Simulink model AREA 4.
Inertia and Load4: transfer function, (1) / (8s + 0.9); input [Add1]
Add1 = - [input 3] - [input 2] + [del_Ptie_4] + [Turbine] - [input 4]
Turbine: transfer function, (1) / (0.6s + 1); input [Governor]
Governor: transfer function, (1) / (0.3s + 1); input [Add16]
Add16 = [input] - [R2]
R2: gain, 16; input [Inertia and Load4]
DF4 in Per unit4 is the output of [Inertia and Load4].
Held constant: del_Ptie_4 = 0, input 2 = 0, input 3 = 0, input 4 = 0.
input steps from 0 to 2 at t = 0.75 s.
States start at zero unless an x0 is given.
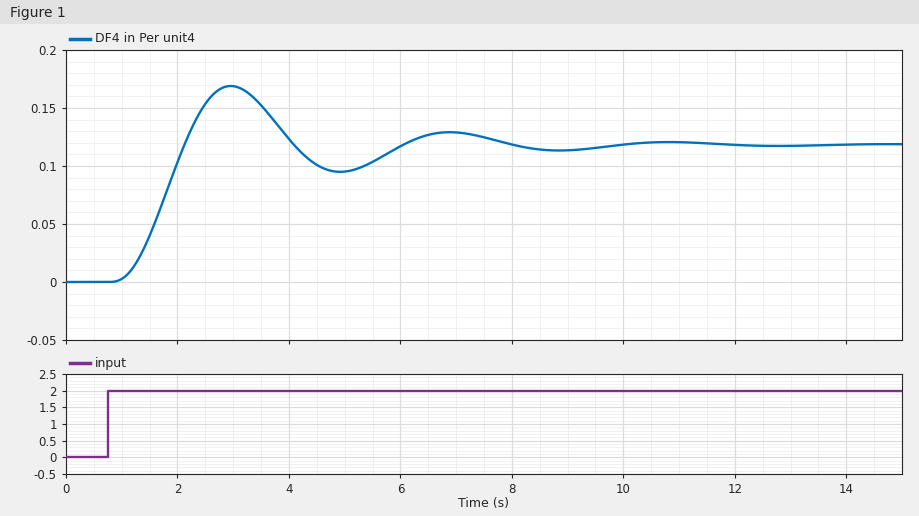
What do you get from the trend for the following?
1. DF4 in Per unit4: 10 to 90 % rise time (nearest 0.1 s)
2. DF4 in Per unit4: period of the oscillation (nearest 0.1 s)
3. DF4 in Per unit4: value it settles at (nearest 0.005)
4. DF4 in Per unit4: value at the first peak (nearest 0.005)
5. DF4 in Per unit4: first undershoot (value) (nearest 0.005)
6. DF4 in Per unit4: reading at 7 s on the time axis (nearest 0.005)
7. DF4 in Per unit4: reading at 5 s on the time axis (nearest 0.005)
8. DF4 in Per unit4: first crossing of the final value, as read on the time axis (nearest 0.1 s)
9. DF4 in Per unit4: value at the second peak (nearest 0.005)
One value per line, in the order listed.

0.8 s
3.9 s
0.120
0.170
0.095
0.130
0.095
2.1 s
0.130
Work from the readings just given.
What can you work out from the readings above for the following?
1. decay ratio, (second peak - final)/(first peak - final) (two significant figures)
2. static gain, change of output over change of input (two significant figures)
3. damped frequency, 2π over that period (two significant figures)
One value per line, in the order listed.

0.20
0.060
1.6 rad/s
